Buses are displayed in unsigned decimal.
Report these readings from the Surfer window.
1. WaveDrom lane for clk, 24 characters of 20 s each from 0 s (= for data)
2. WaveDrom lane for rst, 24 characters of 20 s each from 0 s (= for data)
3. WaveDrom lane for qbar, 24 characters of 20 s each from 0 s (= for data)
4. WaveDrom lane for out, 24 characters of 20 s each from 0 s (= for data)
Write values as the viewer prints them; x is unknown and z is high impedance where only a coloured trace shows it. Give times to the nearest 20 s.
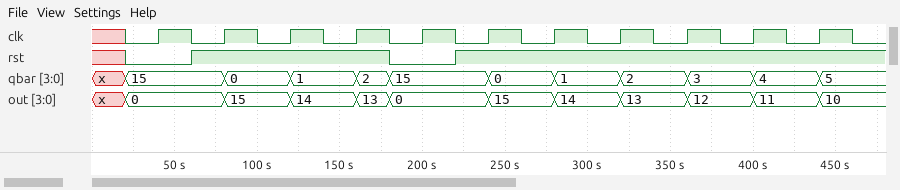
{name: 'clk', wave: 'x01010101010101010101010'}
{name: 'rst', wave: 'x0.1.....0.1............'}
{name: 'qbar', wave: 'x=..=.=.==..=.=.=.=.=.=.', data: '15 0 1 2 15 0 1 2 3 4 5'}
{name: 'out', wave: 'x=..=.=.==..=.=.=.=.=.=.', data: '0 15 14 13 0 15 14 13 12 11 10'}
